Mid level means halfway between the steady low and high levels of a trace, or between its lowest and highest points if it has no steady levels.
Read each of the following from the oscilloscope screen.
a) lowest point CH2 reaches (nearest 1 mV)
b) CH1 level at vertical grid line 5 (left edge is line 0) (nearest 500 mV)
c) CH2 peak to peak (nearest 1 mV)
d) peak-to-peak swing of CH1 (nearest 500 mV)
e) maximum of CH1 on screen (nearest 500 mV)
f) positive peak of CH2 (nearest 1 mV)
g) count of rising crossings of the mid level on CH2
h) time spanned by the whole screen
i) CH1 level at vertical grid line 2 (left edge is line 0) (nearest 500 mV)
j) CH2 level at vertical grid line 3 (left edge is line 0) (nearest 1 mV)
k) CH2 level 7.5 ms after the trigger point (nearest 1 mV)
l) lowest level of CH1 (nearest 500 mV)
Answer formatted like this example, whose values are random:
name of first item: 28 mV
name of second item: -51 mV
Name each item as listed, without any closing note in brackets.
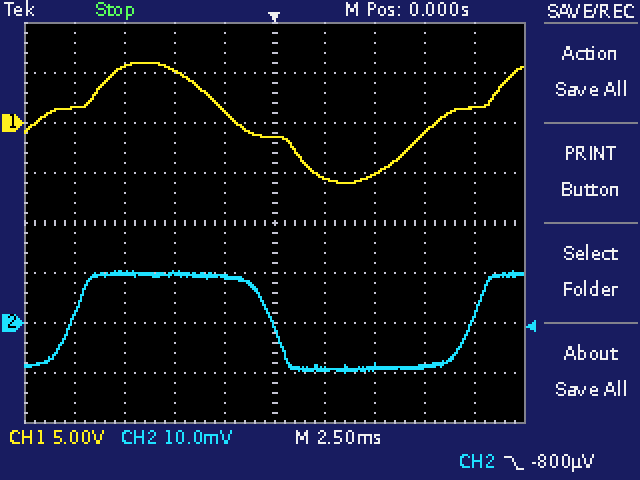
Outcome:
lowest point CH2 reaches: -10 mV
CH1 level at vertical grid line 5 (left edge is line 0): -1.5 V
CH2 peak to peak: 20 mV
peak-to-peak swing of CH1: 12.0 V
maximum of CH1 on screen: 6.0 V
positive peak of CH2: 10 mV
count of rising crossings of the mid level on CH2: 2
time spanned by the whole screen: 25 ms
CH1 level at vertical grid line 2 (left edge is line 0): 5.5 V
CH2 level at vertical grid line 3 (left edge is line 0): 10 mV
CH2 level 7.5 ms after the trigger point: -9 mV
lowest level of CH1: -6.0 V
